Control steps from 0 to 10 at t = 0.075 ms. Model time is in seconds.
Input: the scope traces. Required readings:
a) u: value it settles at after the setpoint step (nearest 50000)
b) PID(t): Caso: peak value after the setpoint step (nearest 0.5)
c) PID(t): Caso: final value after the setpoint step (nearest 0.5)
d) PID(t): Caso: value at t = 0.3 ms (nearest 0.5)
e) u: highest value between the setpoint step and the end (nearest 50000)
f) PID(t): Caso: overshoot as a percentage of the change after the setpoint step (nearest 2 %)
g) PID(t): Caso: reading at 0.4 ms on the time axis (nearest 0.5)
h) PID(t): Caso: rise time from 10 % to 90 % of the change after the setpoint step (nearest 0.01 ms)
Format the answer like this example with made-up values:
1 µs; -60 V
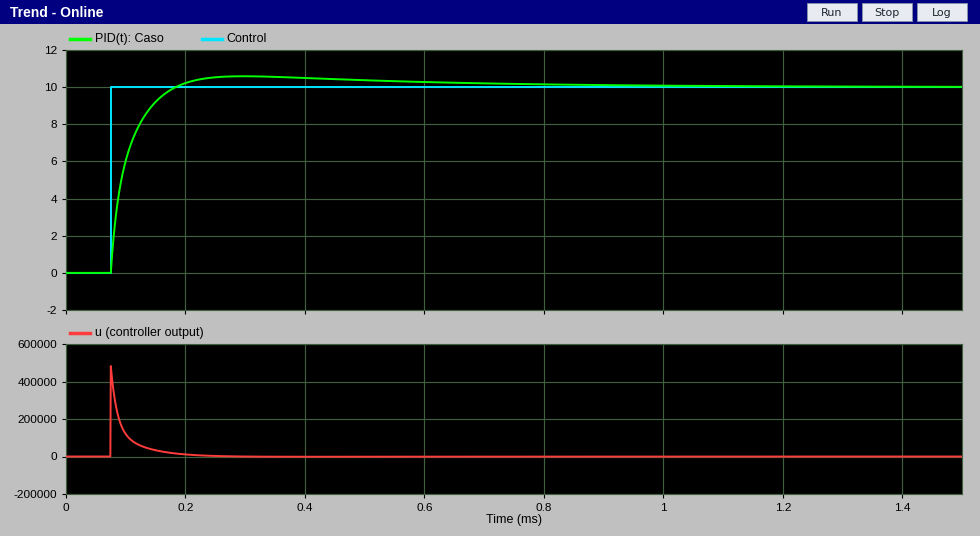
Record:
0; 10.5; 10.0; 10.5; 500000; 6 %; 10.5; 0.07 ms
